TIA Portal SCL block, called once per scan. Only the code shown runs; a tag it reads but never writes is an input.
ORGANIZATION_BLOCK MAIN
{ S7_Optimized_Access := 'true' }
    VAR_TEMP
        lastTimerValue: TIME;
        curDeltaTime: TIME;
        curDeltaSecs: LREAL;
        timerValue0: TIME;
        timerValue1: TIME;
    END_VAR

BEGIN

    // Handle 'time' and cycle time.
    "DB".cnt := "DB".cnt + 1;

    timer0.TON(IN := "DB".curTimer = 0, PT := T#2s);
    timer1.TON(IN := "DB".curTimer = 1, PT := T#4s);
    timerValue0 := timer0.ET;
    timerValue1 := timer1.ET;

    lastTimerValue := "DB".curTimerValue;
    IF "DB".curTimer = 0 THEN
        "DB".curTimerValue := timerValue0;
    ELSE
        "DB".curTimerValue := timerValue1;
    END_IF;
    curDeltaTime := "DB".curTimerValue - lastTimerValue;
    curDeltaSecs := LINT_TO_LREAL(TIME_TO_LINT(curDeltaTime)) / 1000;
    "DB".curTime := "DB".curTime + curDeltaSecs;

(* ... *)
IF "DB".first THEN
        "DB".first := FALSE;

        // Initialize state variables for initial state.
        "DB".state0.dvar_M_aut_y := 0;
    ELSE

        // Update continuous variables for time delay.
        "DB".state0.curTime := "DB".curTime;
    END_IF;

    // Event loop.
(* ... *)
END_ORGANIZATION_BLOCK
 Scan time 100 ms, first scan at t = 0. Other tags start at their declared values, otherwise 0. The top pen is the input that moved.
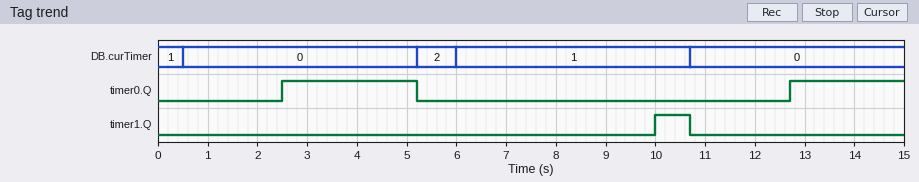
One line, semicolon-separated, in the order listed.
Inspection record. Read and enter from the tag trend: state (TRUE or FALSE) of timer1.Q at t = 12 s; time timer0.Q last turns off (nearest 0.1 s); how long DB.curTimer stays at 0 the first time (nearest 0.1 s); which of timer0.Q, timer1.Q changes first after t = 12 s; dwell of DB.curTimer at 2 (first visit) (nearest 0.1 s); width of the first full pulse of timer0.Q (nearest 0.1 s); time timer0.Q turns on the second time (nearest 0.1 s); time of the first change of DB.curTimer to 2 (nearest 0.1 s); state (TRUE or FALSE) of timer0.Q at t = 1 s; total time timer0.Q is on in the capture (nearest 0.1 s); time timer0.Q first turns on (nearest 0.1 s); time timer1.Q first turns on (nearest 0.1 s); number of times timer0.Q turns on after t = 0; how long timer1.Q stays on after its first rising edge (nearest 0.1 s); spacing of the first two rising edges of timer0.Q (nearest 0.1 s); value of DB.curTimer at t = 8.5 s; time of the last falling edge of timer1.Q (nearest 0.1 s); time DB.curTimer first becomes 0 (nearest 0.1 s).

FALSE; 5.2 s; 4.7 s; timer0.Q; 0.8 s; 2.7 s; 12.7 s; 5.2 s; FALSE; 5.0 s; 2.5 s; 10.0 s; 2; 0.7 s; 10.2 s; 1; 10.7 s; 0.5 s
